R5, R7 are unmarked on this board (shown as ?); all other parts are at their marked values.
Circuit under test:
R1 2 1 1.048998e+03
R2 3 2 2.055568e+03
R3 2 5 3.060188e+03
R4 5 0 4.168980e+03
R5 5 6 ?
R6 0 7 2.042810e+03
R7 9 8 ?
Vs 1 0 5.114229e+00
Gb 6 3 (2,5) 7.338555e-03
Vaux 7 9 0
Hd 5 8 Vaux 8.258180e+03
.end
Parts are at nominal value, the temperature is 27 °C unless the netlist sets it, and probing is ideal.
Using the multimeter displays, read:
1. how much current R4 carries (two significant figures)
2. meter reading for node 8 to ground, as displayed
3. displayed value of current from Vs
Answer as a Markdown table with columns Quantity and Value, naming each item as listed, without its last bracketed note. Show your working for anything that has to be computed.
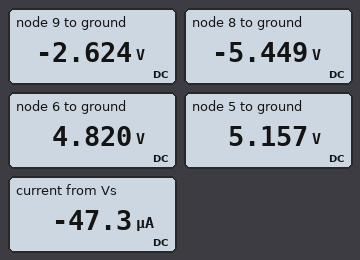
| Quantity | Value |
|---|---|
| how much current R4 carries | (5.157 V) / 4.169 kΩ = 1.2 mA |
| meter reading for node 8 to ground, as displayed | -5.449 V |
| displayed value of current from Vs | -47.3 µA |
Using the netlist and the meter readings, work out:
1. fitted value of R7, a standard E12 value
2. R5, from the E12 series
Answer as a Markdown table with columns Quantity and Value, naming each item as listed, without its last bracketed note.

| Quantity | Value |
|---|---|
| fitted value of R7, a standard E12 value | 2.2 kΩ |
| R5, from the E12 series | 6.8 kΩ |
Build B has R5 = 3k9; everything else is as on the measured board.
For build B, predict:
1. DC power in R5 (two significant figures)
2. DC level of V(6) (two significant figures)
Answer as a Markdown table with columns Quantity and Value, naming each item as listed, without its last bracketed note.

| Quantity | Value |
|---|---|
| DC power in R5 | 9.6 µW |
| DC level of V(6) | 5.0 V |
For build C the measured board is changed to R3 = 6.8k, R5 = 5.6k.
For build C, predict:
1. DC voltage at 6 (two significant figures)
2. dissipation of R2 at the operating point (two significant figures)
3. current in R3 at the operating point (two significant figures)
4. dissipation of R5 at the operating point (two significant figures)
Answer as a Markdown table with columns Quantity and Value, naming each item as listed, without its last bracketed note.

| Quantity | Value |
|---|---|
| DC voltage at 6 | 4.9 V |
| dissipation of R2 at the operating point | 4.8 µW |
| current in R3 at the operating point | 970 nA |
| dissipation of R5 at the operating point | 13 µW |
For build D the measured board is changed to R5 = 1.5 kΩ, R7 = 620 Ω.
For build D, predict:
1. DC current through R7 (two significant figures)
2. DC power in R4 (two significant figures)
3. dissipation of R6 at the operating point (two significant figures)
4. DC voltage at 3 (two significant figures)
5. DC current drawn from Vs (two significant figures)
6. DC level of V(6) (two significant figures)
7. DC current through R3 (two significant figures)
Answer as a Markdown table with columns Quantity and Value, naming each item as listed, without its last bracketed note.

| Quantity | Value |
|---|---|
| DC current through R7 | 870 µA |
| DC power in R4 | 5.6 mW |
| dissipation of R6 at the operating point | 1.5 mW |
| DC voltage at 3 | 4.2 V |
| DC current drawn from Vs | 300 µA |
| DC level of V(6) | 5.3 V |
| DC current through R3 | 14 µA |
